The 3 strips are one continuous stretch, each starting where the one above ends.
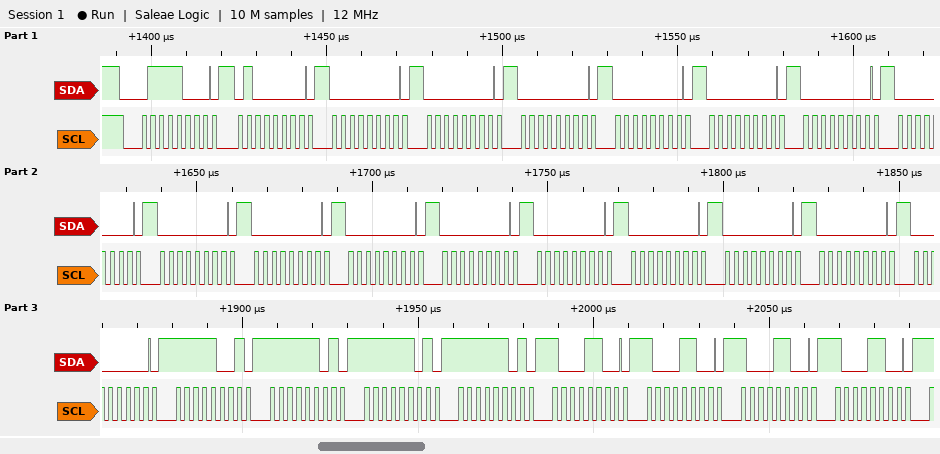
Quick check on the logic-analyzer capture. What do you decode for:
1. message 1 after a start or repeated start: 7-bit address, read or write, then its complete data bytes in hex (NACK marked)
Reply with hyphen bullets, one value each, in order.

- 0x3C write: 40 00 00 00 00 00 00 00 00 00 00 00 00 00 00 00 00 F9 FD FD FD 8C 8C 8C 8C
